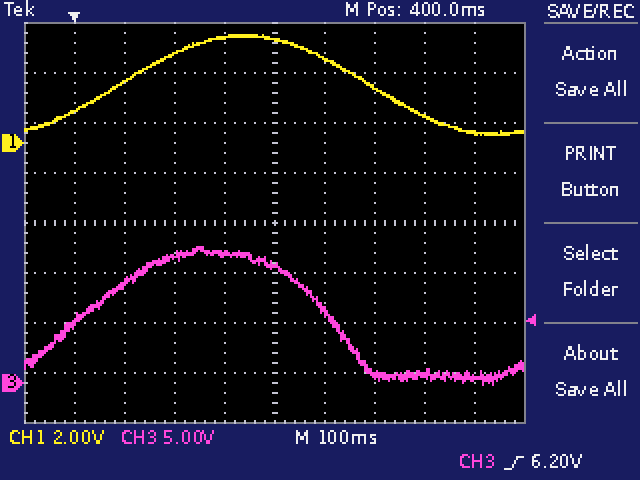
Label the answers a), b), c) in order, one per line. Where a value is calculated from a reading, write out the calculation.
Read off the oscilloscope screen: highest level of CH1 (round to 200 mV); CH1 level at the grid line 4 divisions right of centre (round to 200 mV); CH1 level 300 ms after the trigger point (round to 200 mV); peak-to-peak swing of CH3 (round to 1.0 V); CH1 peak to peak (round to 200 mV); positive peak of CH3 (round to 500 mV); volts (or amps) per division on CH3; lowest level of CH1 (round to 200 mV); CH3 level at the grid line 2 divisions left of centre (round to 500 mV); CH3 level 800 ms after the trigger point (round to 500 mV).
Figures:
a) 4.4 V
b) 400 mV
c) 4.2 V
d) 14.0 V
e) 4.4 V − (400 mV) = 4.0 V
f) 13.5 V
g) 5 V
h) 400 mV
i) 13.0 V
j) 500 mV
